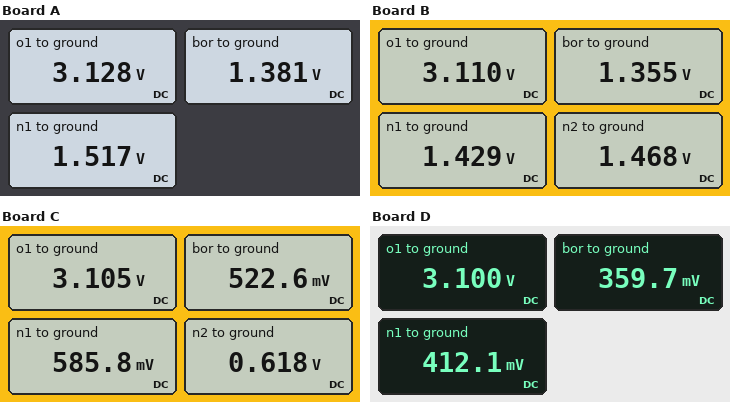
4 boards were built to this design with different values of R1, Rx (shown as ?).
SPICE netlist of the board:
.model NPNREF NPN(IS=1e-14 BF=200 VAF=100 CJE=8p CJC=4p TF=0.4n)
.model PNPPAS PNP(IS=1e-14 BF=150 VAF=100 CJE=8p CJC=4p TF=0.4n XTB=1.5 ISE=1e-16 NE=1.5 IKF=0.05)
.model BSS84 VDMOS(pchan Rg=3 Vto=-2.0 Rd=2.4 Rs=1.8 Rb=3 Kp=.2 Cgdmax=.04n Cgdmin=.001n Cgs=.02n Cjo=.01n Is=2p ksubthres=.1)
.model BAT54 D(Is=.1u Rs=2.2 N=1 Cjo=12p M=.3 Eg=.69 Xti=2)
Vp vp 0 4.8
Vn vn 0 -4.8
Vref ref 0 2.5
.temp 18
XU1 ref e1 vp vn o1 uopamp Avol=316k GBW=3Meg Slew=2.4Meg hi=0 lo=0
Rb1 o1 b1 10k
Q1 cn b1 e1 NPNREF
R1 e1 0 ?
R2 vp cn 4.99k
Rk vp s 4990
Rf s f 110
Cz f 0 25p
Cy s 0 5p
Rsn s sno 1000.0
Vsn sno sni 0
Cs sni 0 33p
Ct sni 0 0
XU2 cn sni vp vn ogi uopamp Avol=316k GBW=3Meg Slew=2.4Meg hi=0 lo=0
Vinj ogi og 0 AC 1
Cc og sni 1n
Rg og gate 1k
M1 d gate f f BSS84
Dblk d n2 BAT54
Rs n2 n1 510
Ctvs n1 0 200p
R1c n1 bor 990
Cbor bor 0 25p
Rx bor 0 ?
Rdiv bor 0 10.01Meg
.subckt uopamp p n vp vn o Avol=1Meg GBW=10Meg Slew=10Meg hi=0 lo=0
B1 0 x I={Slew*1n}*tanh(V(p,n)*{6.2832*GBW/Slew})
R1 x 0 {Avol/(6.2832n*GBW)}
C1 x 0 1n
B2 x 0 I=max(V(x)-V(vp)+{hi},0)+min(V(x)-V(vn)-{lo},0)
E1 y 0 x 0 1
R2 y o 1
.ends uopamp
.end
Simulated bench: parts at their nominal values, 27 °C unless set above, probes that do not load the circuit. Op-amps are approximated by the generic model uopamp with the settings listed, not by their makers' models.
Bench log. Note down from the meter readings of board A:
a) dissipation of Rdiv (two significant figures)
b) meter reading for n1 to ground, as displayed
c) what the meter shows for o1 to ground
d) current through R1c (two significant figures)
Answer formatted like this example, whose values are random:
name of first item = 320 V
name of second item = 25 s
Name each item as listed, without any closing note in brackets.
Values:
dissipation of Rdiv = 190 nW
meter reading for n1 to ground, as displayed = 1.517 V
what the meter shows for o1 to ground = 3.128 V
current through R1c = 140 µA
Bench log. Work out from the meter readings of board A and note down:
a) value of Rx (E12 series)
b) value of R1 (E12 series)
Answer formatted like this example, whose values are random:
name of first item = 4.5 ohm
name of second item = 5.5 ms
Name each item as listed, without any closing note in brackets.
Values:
value of Rx = 10 kΩ
value of R1 = 18 kΩ
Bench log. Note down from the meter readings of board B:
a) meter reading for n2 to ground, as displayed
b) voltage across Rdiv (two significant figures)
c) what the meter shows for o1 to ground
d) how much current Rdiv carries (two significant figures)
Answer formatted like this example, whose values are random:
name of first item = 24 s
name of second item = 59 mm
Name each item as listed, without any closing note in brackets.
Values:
meter reading for n2 to ground, as displayed = 1.468 V
voltage across Rdiv = 1.4 V
what the meter shows for o1 to ground = 3.110 V
how much current Rdiv carries = 140 nA
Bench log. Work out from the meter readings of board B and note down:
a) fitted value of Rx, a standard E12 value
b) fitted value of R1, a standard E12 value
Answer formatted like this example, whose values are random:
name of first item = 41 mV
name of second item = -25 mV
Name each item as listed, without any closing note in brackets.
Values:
fitted value of Rx, a standard E12 value = 18 kΩ
fitted value of R1, a standard E12 value = 33 kΩ
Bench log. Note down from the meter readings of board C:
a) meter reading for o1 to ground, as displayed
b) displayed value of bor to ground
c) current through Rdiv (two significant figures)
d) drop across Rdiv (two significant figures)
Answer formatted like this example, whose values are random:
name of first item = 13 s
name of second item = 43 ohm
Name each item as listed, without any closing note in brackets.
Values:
meter reading for o1 to ground, as displayed = 3.105 V
displayed value of bor to ground = 522.6 mV
current through Rdiv = 52 nA
drop across Rdiv = 520 mV
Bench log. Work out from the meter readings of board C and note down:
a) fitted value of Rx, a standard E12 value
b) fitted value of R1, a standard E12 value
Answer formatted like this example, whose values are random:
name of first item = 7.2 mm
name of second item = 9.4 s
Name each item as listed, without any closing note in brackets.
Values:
fitted value of Rx, a standard E12 value = 8.2 kΩ
fitted value of R1, a standard E12 value = 39 kΩ
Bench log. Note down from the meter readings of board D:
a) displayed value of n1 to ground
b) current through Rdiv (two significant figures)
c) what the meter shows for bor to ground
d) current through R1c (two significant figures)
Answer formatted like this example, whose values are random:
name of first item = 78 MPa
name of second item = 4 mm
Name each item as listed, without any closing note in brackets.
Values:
displayed value of n1 to ground = 412.1 mV
current through Rdiv = 36 nA
what the meter shows for bor to ground = 359.7 mV
current through R1c = 53 µA
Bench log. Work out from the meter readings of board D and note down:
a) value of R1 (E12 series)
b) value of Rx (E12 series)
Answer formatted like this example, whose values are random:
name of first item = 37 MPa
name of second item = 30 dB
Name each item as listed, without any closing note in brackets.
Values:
value of R1 = 47 kΩ
value of Rx = 6.8 kΩ
